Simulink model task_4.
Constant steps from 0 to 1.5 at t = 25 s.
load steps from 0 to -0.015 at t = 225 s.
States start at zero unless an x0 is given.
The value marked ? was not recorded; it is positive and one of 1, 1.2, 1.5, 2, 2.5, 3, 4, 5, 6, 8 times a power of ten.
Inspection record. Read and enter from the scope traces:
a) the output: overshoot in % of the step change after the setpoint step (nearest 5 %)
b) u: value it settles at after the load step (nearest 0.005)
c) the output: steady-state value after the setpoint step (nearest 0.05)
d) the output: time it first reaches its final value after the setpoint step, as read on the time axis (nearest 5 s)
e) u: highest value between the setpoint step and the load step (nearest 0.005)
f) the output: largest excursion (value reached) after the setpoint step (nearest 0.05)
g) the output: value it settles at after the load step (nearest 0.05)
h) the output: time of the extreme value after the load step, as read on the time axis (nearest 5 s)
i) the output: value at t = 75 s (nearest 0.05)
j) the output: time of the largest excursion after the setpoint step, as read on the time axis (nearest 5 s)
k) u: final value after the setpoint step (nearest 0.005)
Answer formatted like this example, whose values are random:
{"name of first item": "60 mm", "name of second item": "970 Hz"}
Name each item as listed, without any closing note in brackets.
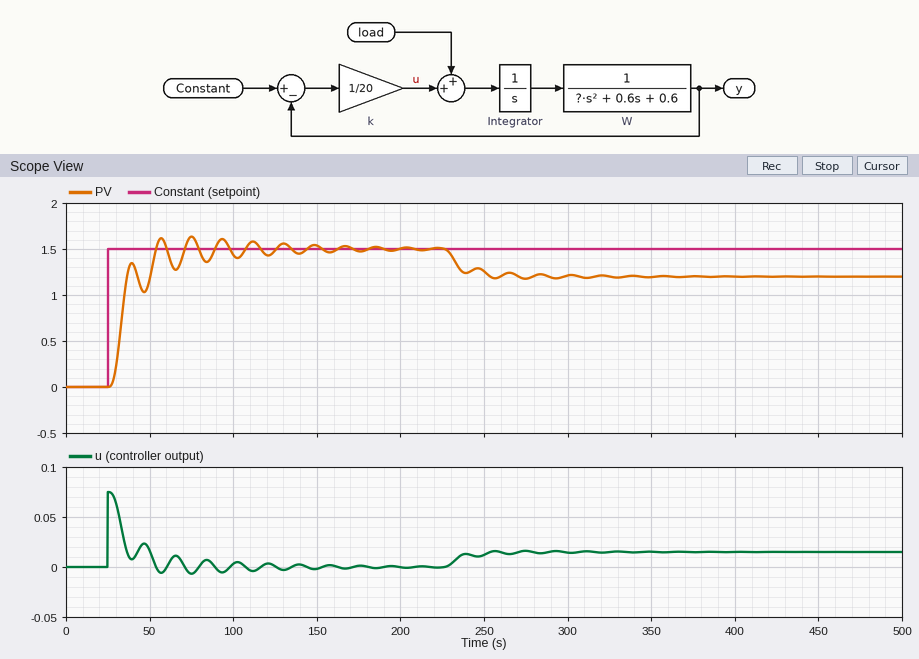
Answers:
{"the output: overshoot in % of the step change after the setpoint step": "10 %", "u: value it settles at after the load step": "0.015", "the output: steady-state value after the setpoint step": "1.50", "the output: time it first reaches its final value after the setpoint step, as read on the time axis": "55 s", "u: highest value between the setpoint step and the load step": "0.075", "the output: largest excursion (value reached) after the setpoint step": "1.65", "the output: value it settles at after the load step": "1.20", "the output: time of the extreme value after the load step, as read on the time axis": "275 s", "the output: value at t = 75 s": "1.65", "the output: time of the largest excursion after the setpoint step, as read on the time axis": "75 s", "u: final value after the setpoint step": "0.000"}
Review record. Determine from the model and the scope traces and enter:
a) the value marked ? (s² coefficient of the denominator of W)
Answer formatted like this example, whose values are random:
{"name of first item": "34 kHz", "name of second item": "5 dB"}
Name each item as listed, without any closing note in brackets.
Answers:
{"the value marked ?": "5"}
